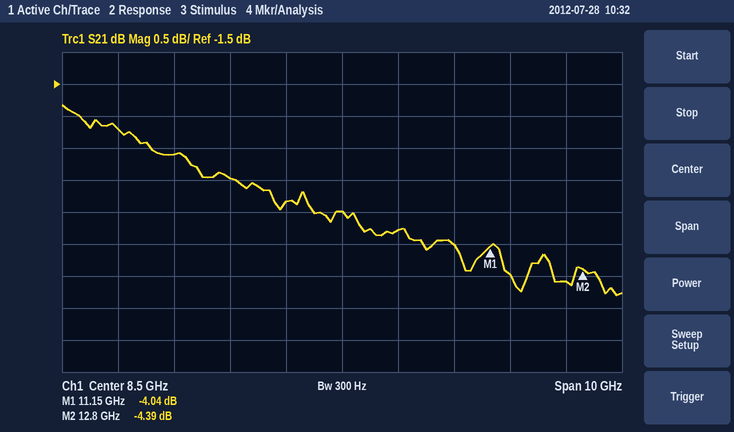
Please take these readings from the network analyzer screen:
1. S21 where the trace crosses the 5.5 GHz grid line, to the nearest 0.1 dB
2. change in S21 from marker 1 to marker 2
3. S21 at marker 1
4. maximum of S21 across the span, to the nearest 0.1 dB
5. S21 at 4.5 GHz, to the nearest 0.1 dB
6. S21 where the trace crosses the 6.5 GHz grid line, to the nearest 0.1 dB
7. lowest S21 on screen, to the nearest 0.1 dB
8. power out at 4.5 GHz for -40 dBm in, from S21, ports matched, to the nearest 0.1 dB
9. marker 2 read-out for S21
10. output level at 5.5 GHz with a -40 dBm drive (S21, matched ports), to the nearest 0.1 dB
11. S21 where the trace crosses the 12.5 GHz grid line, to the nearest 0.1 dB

-2.6 dB
-0.35 dB
-4.04 dB
-1.8 dB
-2.2 dB
-3.0 dB
-4.8 dB
-42.2 dBm
-4.39 dB
-42.6 dBm
-4.6 dB
